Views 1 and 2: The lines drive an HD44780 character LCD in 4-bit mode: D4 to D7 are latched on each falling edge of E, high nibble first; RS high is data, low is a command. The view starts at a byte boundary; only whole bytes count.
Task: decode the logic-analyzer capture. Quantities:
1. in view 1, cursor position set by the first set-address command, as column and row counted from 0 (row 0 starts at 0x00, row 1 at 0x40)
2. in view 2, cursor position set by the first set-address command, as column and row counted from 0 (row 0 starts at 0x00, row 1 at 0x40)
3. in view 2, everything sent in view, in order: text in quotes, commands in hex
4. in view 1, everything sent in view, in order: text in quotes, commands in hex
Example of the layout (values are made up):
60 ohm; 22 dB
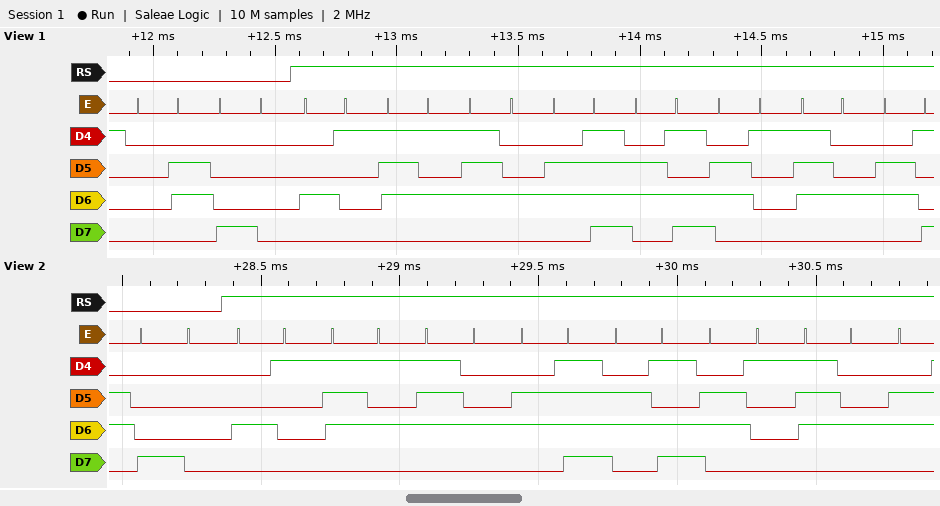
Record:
column 0, row 0; column 0, row 0; 0x80 "Automat"; 0x06 0x80 "Automati"
